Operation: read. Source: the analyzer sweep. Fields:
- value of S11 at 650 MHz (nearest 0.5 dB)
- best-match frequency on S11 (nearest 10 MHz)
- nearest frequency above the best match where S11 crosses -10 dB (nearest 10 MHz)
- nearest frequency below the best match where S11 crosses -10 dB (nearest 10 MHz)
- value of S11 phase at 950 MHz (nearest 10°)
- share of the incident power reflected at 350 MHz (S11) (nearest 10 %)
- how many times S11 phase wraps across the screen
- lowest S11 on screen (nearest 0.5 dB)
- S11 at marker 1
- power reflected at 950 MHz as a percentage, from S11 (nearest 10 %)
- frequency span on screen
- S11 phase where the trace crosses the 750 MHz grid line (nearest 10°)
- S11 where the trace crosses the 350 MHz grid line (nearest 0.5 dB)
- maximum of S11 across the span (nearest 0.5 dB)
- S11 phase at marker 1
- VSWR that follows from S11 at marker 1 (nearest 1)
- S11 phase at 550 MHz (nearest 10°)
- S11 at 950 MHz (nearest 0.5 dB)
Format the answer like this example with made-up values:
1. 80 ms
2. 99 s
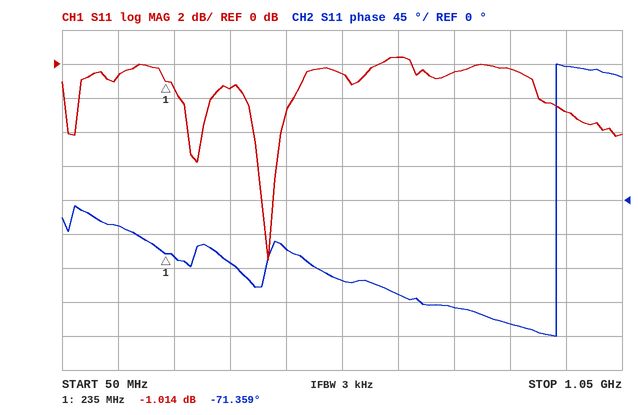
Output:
1. 0.5 dB
2. 420 MHz
3. 420 MHz
4. 410 MHz
5. 180°
6. 70 %
7. 1
8. -11.5 dB
9. -1.014 dB
10. 50 %
11. 1 GHz
12. -140°
13. -1.5 dB
14. 0.5 dB
15. -71.359°
16. 17
17. -110°
18. -3.0 dB
